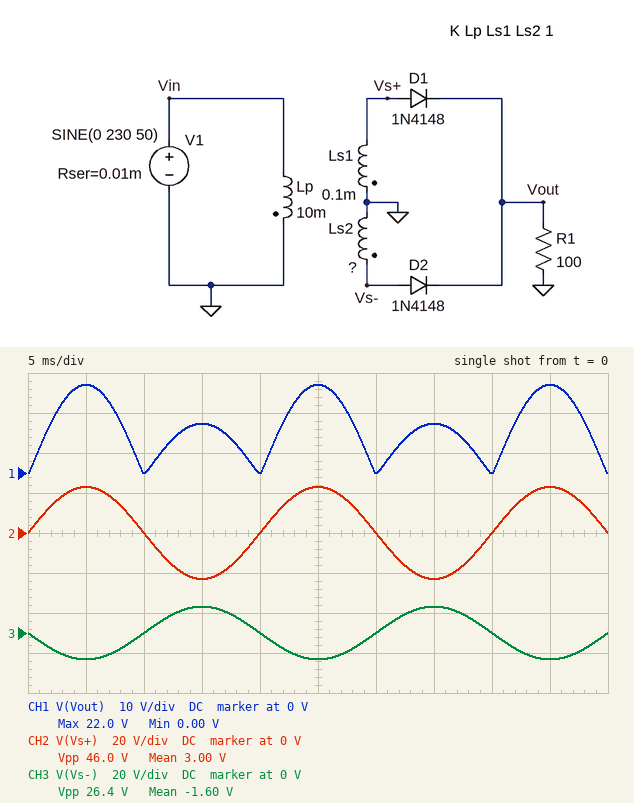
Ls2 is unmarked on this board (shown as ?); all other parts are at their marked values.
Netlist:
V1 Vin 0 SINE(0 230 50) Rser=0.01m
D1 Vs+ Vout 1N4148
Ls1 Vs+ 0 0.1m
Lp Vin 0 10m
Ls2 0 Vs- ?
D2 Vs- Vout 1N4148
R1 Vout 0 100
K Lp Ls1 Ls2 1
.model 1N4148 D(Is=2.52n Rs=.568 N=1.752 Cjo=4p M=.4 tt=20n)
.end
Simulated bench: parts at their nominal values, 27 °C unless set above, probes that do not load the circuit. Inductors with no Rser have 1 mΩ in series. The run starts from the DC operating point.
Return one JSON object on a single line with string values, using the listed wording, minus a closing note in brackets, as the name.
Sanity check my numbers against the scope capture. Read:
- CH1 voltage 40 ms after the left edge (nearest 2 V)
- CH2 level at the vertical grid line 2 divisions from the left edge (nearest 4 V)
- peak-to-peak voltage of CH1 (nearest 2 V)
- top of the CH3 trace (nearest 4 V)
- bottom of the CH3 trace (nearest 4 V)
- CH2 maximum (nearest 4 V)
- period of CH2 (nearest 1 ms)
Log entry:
{"CH1 voltage 40 ms after the left edge": "0 V", "CH2 level at the vertical grid line 2 divisions from the left edge": "0 V", "peak-to-peak voltage of CH1": "22 V", "top of the CH3 trace": "12 V", "bottom of the CH3 trace": "-12 V", "CH2 maximum": "24 V", "period of CH2": "20 ms"}
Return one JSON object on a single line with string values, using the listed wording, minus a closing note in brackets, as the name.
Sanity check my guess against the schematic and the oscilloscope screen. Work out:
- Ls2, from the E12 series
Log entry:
{"Ls2, from the E12 series": "33 µH"}
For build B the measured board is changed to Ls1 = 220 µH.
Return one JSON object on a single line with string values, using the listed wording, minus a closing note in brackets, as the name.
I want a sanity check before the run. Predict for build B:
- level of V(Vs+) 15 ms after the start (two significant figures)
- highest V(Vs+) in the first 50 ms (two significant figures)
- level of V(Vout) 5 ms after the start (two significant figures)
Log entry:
{"level of V(Vs+) 15 ms after the start": "-34 V", "highest V(Vs+) in the first 50 ms": "34 V", "level of V(Vout) 5 ms after the start": "33 V"}
